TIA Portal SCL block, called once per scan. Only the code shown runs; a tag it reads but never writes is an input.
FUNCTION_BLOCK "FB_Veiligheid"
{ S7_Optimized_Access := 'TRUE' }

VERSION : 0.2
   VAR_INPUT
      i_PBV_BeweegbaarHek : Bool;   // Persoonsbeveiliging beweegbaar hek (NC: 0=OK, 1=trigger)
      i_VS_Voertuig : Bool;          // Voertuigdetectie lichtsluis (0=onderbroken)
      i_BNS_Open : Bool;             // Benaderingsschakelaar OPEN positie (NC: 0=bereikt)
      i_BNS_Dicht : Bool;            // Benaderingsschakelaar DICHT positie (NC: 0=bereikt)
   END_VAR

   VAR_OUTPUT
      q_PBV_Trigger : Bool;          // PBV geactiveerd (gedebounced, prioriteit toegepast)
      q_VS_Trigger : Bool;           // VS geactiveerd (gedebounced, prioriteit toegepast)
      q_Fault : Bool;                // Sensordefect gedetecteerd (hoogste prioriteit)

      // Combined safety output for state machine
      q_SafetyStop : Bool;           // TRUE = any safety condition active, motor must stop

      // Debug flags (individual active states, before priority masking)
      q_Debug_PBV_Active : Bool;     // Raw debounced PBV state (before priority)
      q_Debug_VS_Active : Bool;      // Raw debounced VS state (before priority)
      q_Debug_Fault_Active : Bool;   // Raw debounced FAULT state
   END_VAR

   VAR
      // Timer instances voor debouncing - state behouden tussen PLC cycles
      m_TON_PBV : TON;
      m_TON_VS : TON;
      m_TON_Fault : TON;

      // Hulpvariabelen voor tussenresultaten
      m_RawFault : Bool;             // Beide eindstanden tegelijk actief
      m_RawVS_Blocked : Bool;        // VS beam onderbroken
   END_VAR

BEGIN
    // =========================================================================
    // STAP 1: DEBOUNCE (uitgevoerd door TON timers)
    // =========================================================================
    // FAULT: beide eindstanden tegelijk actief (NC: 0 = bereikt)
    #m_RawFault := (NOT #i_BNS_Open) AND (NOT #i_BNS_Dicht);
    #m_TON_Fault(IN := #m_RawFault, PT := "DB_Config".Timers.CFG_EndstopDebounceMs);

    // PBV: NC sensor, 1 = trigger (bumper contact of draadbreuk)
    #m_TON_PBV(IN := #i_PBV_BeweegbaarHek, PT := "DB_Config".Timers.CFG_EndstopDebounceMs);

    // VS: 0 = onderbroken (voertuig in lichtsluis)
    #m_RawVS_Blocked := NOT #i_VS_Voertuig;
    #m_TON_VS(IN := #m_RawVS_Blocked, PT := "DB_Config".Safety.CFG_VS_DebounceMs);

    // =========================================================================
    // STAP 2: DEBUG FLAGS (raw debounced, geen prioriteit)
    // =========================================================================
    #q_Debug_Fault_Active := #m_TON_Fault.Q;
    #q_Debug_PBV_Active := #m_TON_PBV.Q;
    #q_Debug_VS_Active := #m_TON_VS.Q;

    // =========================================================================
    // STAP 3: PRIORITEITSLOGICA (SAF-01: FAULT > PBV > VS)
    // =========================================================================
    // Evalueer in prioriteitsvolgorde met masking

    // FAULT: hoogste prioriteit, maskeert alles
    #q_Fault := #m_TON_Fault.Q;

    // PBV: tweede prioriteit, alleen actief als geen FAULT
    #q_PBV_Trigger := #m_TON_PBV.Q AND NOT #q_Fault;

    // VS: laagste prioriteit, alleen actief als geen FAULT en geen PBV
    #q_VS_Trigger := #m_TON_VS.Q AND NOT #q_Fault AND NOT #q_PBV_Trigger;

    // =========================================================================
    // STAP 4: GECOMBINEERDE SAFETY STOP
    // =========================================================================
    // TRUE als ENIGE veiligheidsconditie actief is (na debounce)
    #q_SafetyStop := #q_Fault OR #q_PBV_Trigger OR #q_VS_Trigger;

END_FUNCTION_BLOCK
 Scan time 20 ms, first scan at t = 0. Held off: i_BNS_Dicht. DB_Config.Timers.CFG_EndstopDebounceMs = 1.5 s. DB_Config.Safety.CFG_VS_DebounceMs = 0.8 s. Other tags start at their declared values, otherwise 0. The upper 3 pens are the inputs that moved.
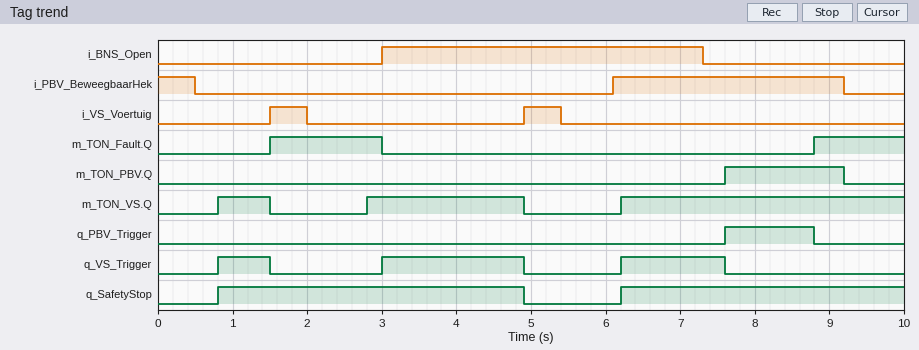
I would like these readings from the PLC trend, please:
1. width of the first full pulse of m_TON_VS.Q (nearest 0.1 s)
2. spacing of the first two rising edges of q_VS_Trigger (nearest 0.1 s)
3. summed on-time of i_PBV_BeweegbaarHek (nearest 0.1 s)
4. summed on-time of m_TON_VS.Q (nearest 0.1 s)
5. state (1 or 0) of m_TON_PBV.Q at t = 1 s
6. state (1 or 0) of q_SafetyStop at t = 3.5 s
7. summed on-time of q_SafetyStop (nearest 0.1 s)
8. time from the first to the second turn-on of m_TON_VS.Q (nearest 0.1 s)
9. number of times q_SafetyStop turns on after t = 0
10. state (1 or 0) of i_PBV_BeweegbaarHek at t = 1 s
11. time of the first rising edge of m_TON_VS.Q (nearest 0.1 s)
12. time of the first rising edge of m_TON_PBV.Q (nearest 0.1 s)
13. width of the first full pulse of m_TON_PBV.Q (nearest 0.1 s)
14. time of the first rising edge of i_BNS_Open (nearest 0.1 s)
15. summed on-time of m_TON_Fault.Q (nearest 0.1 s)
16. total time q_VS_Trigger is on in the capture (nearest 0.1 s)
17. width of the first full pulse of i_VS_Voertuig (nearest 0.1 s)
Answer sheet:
0.7 s
2.2 s
3.6 s
6.6 s
0
1
7.9 s
2.0 s
2
0
0.8 s
7.6 s
1.6 s
3.0 s
2.7 s
4.0 s
0.5 s
